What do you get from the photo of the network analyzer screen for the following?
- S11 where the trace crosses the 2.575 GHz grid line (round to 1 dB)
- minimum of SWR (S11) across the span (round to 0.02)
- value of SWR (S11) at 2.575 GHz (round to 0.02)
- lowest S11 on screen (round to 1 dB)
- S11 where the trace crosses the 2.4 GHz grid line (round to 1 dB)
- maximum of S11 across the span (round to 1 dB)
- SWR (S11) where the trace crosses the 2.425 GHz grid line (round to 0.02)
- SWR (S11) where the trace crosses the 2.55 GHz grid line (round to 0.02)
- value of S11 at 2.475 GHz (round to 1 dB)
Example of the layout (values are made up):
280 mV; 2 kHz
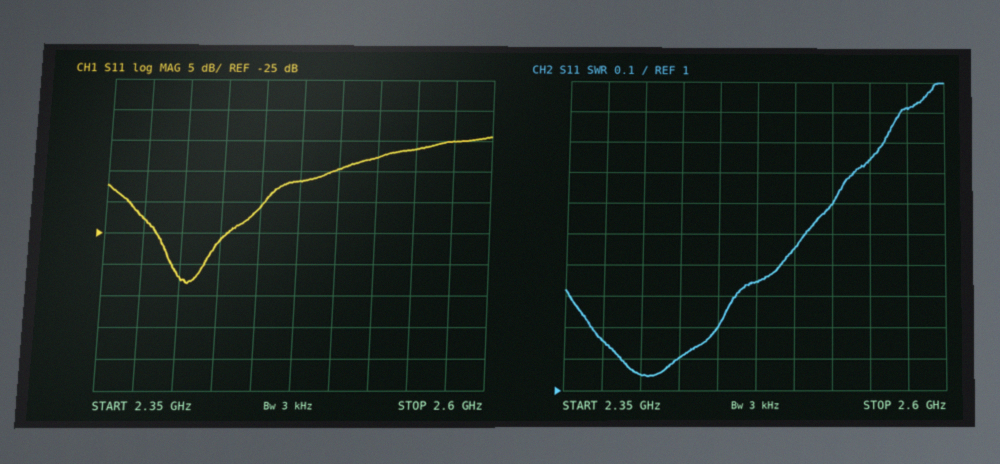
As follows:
-10 dB; 1.04; 1.92; -33 dB; -32 dB; -9 dB; 1.10; 1.74; -17 dB
